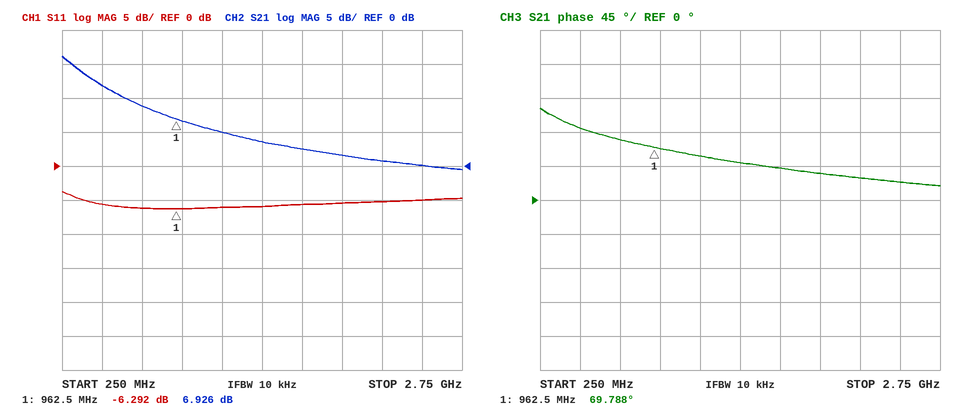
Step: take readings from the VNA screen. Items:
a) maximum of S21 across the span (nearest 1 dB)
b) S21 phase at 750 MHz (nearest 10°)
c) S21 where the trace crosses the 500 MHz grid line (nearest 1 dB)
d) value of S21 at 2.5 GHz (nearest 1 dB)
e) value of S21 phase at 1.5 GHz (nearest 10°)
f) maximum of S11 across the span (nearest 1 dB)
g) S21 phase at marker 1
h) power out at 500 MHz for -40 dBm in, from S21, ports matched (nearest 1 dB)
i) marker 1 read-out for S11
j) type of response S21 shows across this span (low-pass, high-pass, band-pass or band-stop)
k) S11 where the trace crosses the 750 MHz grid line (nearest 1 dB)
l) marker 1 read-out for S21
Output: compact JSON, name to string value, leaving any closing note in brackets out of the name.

{"maximum of S21 across the span": "16 dB", "S21 phase at 750 MHz": "80°", "S21 where the trace crosses the 500 MHz grid line": "12 dB", "value of S21 at 2.5 GHz": "0 dB", "value of S21 phase at 1.5 GHz": "50°", "maximum of S11 across the span": "-4 dB", "S21 phase at marker 1": "69.788°", "power out at 500 MHz for -40 dBm in, from S21, ports matched": "-28 dBm", "marker 1 read-out for S11": "-6.292 dB", "type of response S21 shows across this span": "low-pass", "S11 where the trace crosses the 750 MHz grid line": "-6 dB", "marker 1 read-out for S21": "6.926 dB"}
